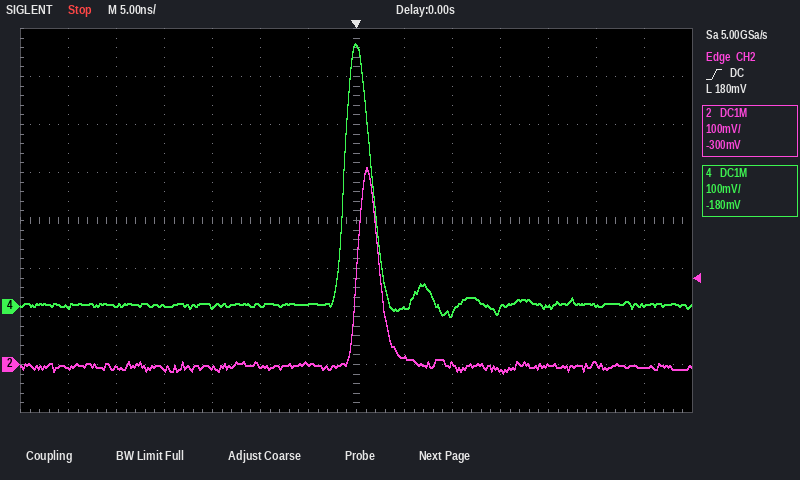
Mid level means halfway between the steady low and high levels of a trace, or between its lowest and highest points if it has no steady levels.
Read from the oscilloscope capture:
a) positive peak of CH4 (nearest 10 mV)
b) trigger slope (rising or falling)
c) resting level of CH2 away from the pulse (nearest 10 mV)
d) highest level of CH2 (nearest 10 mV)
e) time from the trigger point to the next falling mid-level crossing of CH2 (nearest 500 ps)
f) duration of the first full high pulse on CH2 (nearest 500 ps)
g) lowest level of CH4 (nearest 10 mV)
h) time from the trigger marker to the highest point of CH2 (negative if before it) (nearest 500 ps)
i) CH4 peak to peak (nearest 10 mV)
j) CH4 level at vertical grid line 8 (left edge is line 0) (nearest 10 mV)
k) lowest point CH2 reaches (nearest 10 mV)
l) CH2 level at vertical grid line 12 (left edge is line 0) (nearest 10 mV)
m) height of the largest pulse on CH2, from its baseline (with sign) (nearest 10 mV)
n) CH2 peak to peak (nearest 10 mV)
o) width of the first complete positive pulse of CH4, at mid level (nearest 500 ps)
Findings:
550 mV
rising
0 mV
410 mV
2.5 ns
2.5 ns
-20 mV
+1.0 ns
570 mV
0 mV
-20 mV
0 mV
+410 mV
430 mV
3.0 ns
